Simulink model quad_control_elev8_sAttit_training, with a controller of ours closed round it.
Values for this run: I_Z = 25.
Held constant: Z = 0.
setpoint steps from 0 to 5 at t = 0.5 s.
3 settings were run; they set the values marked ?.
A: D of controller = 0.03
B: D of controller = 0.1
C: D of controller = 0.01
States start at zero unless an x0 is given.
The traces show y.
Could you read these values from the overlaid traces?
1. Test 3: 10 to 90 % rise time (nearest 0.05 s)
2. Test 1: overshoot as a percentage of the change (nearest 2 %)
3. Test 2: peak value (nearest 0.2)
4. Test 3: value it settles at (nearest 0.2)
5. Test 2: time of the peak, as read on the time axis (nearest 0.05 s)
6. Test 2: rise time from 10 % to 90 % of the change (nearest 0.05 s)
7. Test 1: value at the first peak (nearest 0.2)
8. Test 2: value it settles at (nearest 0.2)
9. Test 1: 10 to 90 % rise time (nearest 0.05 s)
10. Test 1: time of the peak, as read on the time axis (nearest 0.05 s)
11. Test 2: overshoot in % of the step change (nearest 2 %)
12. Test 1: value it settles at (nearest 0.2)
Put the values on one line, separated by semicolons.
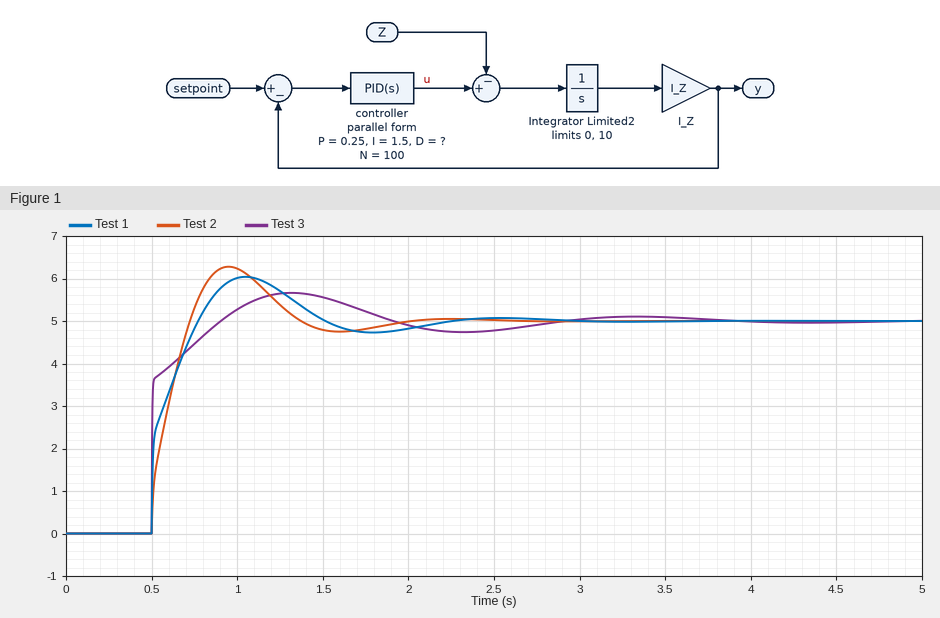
0.25 s; 20 %; 6.2; 5.0; 0.95 s; 0.20 s; 6.0; 5.0; 0.20 s; 1.05 s; 26 %; 5.0
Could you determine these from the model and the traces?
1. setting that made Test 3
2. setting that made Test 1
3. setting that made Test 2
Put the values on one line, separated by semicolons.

B; A; C
